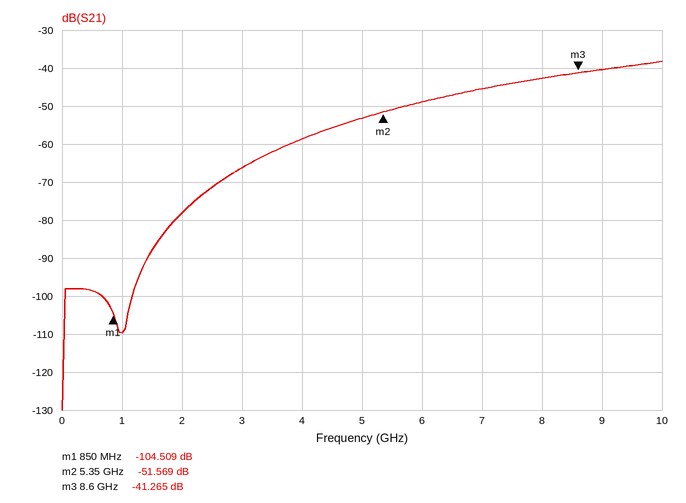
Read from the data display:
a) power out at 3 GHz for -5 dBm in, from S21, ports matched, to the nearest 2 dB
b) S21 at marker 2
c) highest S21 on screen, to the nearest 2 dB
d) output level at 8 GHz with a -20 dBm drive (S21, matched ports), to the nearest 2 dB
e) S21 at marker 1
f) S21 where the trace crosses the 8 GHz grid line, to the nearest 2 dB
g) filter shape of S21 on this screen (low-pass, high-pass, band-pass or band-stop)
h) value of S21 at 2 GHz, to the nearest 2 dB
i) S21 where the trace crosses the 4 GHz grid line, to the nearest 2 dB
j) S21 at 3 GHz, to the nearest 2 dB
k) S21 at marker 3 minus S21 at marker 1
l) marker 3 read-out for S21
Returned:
-72 dBm
-51.569 dB
-38 dB
-62 dBm
-104.509 dB
-42 dB
high-pass
-78 dB
-58 dB
-66 dB
63.244 dB
-41.265 dB
